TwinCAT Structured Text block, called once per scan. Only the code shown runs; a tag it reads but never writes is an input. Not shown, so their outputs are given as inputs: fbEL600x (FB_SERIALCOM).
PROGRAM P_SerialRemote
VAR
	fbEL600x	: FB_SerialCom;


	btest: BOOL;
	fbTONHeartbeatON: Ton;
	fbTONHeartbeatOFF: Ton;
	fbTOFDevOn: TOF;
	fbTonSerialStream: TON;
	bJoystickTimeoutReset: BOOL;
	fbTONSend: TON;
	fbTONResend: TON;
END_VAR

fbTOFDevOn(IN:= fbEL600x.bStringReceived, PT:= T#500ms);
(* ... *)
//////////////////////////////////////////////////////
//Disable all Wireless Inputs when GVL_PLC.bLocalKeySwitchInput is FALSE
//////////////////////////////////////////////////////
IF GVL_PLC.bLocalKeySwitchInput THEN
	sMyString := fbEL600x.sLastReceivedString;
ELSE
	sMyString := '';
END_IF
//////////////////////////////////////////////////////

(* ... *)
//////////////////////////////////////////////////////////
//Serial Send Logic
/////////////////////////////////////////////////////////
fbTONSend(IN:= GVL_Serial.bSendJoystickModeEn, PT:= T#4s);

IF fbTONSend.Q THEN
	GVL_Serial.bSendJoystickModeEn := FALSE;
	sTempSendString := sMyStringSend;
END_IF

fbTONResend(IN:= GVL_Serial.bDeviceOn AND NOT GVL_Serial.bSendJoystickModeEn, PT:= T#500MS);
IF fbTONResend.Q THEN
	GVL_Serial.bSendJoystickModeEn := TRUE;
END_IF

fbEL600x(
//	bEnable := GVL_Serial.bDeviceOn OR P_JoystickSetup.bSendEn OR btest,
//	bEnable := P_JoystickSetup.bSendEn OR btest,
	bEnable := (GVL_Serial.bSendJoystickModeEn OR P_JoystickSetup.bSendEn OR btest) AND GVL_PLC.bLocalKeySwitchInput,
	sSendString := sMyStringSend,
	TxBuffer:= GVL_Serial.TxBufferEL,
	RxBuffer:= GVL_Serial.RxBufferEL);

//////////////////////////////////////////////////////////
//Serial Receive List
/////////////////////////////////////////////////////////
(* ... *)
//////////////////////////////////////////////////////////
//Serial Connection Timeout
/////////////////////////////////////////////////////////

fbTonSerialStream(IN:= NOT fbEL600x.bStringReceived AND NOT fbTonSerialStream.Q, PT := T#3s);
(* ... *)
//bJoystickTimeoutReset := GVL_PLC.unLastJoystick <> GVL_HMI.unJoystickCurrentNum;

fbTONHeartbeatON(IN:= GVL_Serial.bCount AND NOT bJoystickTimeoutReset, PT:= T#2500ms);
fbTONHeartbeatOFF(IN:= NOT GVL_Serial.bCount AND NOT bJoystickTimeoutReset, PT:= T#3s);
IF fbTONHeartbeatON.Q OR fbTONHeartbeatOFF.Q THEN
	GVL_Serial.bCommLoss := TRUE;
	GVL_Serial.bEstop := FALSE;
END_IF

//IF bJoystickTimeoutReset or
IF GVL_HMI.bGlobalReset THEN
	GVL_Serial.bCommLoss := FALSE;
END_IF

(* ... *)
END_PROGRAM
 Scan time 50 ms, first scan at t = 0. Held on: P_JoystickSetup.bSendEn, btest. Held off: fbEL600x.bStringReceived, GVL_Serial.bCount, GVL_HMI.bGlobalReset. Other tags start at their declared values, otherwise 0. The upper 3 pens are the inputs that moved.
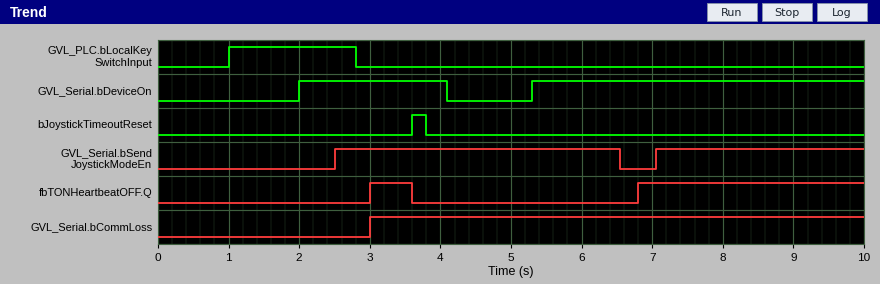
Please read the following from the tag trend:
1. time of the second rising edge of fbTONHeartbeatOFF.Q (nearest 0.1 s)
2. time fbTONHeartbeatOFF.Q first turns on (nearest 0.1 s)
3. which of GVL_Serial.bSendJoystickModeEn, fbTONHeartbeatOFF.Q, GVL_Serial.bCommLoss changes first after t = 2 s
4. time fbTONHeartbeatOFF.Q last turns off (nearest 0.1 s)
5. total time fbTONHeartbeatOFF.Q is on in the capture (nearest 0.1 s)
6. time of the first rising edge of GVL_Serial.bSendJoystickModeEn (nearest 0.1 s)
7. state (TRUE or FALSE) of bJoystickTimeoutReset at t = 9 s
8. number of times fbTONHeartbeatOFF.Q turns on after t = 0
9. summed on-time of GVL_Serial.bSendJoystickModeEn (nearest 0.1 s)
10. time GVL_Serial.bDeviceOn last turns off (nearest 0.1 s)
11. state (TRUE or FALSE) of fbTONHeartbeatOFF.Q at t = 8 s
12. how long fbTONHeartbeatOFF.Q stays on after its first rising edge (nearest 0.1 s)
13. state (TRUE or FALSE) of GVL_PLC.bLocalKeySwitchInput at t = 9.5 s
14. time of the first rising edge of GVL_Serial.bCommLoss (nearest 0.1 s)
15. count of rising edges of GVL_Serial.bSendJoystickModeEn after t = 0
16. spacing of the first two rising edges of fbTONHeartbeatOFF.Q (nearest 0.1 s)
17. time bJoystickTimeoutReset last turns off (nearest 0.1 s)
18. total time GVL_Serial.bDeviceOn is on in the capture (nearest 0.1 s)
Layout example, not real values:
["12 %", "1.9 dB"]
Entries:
["6.8 s", "3.0 s", "GVL_Serial.bSendJoystickModeEn", "3.6 s", "3.8 s", "2.5 s", "FALSE", "2", "7.0 s", "4.1 s", "TRUE", "0.6 s", "FALSE", "3.0 s", "2", "3.8 s", "3.8 s", "6.8 s"]
